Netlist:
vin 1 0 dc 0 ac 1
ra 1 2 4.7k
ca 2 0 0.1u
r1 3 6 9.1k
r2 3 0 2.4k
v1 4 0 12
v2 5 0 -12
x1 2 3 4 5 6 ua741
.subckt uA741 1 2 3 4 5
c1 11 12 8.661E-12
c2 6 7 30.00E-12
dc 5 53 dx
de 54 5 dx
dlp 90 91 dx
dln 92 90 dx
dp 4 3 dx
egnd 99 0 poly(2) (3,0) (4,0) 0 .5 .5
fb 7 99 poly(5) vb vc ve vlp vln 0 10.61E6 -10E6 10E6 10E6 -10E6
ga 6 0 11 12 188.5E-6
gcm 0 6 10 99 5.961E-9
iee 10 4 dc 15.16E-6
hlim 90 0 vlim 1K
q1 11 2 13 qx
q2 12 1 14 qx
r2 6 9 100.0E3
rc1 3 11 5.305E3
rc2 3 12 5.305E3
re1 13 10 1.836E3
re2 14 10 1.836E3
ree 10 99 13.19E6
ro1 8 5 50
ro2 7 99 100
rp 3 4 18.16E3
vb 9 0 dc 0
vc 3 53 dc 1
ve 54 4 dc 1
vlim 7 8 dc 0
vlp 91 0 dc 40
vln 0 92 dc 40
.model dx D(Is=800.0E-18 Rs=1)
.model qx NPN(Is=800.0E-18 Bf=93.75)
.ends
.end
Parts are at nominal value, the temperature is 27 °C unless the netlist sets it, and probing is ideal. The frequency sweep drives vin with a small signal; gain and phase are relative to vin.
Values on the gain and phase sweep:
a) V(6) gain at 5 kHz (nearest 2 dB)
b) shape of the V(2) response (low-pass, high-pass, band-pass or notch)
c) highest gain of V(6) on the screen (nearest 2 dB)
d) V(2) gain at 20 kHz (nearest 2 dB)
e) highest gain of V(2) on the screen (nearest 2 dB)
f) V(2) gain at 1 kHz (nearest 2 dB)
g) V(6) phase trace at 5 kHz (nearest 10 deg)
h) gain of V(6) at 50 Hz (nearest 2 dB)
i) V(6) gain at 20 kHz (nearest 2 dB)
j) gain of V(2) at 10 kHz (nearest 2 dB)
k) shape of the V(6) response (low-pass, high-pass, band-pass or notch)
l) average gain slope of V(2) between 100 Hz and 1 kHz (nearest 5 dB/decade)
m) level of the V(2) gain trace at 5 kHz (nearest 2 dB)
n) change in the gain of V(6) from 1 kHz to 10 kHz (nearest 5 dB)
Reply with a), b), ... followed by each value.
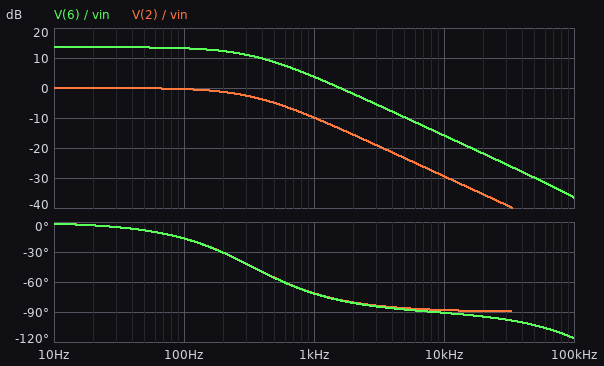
a) -10 dB
b) low-pass
c) 14 dB
d) -36 dB
e) 0 dB
f) -10 dB
g) -90 deg
h) 14 dB
i) -22 dB
j) -30 dB
k) low-pass
l) -10 dB/decade
m) -24 dB
n) -20 dB
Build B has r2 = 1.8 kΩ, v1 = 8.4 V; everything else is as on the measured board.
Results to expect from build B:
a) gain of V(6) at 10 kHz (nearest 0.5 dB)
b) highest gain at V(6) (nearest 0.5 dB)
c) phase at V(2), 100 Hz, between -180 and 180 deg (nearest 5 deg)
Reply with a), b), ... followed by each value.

a) -14.0 dB
b) 15.5 dB
c) -15 deg
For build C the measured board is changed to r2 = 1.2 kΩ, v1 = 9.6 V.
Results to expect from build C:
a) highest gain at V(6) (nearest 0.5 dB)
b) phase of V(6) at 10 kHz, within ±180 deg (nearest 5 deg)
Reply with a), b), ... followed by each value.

a) 18.5 dB
b) -95 deg
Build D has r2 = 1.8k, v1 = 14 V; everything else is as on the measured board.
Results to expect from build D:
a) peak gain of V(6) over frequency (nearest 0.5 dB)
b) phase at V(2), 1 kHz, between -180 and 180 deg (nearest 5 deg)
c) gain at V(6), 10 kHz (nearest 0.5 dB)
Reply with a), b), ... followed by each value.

a) 15.5 dB
b) -70 deg
c) -14.0 dB
